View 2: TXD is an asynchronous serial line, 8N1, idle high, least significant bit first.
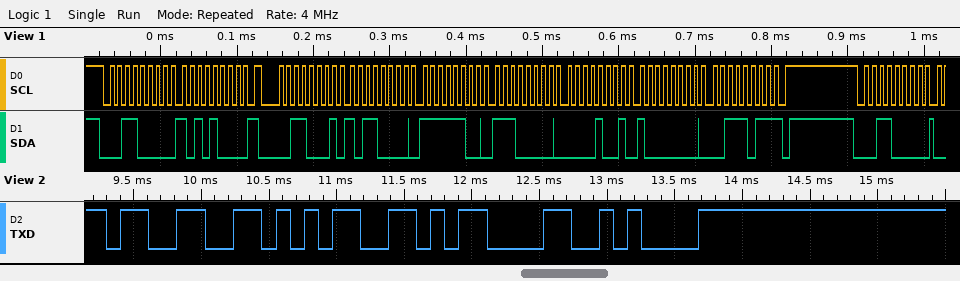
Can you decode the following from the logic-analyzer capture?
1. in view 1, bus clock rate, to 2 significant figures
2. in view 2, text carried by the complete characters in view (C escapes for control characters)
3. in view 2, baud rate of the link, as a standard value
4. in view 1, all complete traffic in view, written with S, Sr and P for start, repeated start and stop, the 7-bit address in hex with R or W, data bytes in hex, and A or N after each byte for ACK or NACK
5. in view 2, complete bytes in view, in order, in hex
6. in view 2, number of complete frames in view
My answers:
100 kHz
"35\r\n"
9600 baud
S 18W A A8 A Sr 18R A B0 A FC A E0 A 09 A 80 A 3B N P S 18W A
0x33 0x35 0x0D 0x0A
4
